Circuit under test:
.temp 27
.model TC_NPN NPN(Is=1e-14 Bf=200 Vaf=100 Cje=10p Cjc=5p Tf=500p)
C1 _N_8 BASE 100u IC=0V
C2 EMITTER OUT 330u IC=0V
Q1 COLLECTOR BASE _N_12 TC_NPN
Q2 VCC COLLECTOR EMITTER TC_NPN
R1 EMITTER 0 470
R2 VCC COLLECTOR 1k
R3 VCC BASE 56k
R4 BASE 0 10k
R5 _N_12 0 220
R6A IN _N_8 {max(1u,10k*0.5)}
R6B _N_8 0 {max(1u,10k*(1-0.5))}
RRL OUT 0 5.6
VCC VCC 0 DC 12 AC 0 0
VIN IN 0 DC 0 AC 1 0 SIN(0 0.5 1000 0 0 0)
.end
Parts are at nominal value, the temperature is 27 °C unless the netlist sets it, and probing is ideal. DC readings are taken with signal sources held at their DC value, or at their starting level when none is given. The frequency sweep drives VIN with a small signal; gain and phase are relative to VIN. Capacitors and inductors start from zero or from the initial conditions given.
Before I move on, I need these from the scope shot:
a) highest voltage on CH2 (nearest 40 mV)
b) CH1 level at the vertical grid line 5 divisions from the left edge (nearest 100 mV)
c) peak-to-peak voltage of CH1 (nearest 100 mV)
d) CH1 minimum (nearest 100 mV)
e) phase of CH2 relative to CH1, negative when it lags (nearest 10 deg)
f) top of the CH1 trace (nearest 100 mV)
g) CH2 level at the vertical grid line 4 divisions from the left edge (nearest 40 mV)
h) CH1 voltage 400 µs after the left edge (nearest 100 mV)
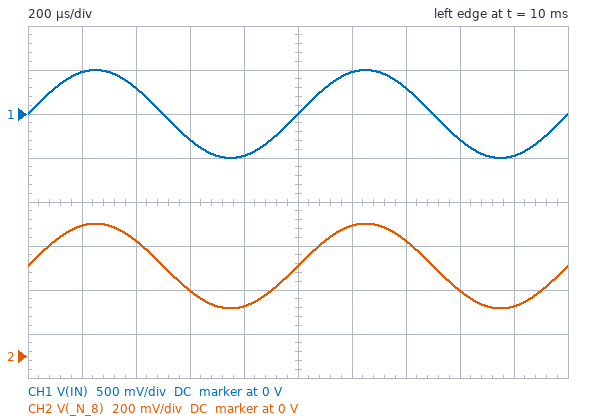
600 mV
0 V
1.0 V
-500 mV
0 deg
500 mV
240 mV
300 mV
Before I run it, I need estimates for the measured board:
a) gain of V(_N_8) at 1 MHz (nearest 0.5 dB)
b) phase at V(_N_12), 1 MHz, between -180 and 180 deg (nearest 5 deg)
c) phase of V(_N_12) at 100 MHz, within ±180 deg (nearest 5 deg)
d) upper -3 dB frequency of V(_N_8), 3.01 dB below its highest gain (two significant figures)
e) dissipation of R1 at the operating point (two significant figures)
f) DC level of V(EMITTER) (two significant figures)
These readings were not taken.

-9.0 dB
-5 deg
-65 deg
10 MHz
100 mW
6.9 V
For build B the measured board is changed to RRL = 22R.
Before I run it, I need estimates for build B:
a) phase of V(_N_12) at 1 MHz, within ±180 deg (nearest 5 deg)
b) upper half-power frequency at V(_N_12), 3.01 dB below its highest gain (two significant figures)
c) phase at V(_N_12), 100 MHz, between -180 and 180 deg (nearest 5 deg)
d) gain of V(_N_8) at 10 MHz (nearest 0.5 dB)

-10 deg
5.2 MHz
-60 deg
-13.5 dB
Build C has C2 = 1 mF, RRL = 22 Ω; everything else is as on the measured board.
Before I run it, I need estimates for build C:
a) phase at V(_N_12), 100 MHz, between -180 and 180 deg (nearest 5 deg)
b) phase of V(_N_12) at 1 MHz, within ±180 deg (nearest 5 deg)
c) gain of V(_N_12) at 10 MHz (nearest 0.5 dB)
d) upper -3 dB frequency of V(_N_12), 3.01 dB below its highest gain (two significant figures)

-60 deg
-10 deg
-13.5 dB
5.2 MHz
